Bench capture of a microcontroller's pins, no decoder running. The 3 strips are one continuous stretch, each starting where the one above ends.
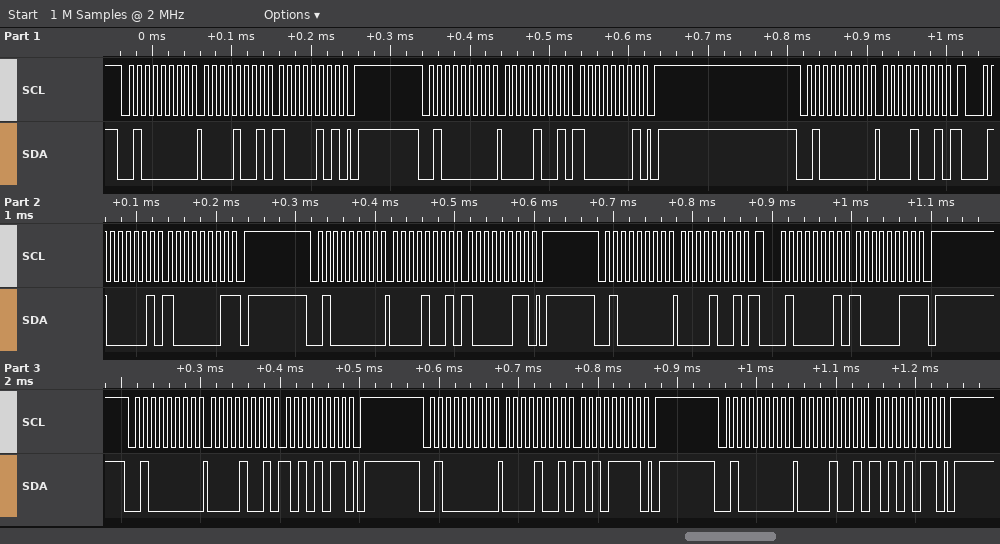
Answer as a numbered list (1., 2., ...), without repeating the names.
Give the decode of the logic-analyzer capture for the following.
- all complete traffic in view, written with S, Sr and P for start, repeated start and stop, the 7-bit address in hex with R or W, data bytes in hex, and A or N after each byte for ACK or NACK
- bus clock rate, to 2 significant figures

1. S 20W A 09 A 85 A P S 20W A 09 A 81 A P S 20W A 09 A Sr 20R A 81 N P S 20W A 09 A 83 A P S 20W A 09 A Sr 20R A 83 N P S 20W A 09 A AB A P S 20W A 09 A AF A P S 20W A 09 A AB A P
2. 100 kHz
